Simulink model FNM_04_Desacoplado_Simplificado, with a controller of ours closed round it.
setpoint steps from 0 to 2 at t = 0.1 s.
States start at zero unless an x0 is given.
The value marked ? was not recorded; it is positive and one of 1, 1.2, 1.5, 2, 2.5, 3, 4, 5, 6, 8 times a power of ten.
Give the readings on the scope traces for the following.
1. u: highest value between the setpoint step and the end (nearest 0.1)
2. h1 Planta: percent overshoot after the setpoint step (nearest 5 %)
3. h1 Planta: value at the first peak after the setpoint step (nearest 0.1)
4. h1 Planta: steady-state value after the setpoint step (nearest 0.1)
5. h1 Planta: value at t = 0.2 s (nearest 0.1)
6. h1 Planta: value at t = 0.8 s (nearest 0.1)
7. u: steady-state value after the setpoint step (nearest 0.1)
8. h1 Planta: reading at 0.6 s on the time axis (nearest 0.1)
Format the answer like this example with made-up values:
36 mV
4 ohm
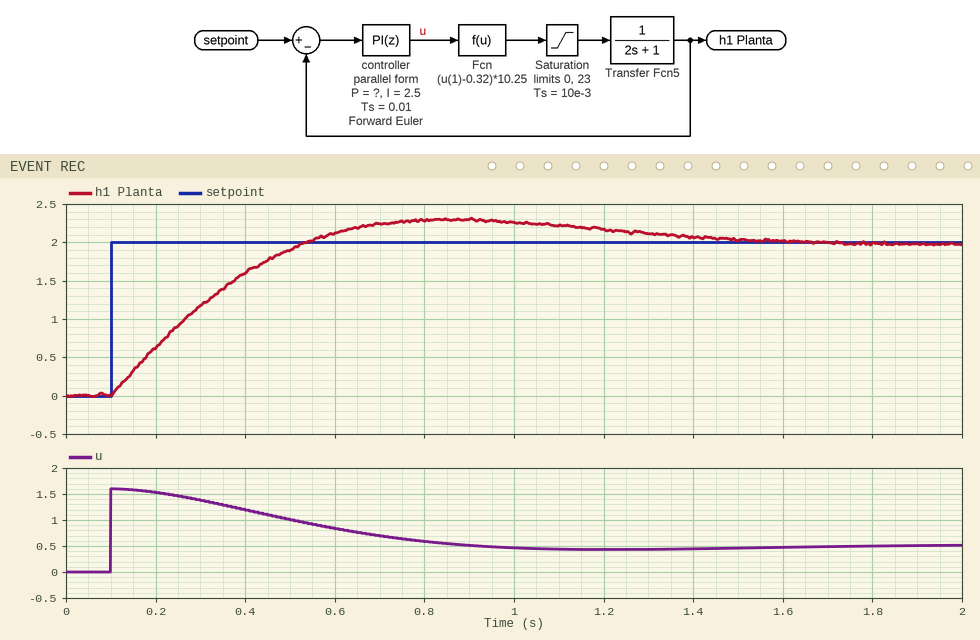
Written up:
1.6
15 %
2.3
2.0
0.6
2.3
0.5
2.1
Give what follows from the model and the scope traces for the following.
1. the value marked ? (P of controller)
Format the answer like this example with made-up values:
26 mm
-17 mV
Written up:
0.8
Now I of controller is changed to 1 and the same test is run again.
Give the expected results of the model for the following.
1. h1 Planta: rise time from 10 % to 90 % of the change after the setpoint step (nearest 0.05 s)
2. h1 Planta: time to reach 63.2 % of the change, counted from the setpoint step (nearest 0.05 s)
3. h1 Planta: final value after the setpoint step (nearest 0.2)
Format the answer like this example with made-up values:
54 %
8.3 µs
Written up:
0.60 s
0.30 s
2.0
